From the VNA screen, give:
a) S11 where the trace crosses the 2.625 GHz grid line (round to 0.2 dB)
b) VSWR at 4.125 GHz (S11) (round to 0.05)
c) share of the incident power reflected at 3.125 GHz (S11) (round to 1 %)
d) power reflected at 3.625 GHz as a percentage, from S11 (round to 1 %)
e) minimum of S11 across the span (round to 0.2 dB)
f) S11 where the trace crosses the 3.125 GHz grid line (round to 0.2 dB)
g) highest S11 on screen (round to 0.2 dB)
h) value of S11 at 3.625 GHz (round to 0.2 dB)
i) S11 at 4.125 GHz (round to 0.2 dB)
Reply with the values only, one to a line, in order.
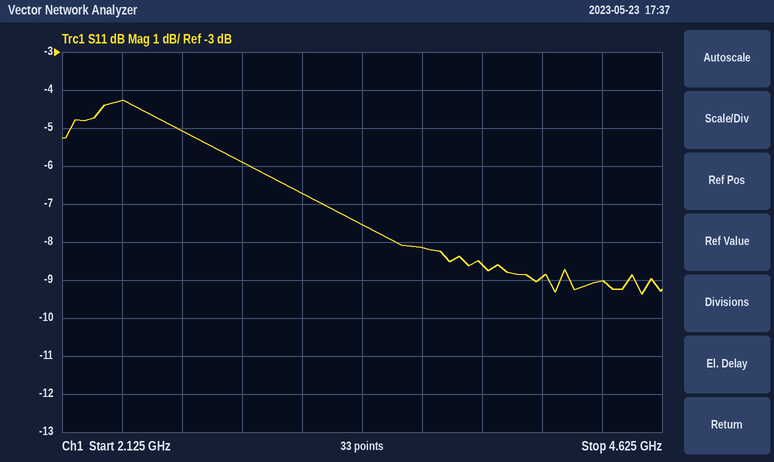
-5.0 dB
2.10
21 %
15 %
-9.4 dB
-6.8 dB
-4.2 dB
-8.2 dB
-9.0 dB
